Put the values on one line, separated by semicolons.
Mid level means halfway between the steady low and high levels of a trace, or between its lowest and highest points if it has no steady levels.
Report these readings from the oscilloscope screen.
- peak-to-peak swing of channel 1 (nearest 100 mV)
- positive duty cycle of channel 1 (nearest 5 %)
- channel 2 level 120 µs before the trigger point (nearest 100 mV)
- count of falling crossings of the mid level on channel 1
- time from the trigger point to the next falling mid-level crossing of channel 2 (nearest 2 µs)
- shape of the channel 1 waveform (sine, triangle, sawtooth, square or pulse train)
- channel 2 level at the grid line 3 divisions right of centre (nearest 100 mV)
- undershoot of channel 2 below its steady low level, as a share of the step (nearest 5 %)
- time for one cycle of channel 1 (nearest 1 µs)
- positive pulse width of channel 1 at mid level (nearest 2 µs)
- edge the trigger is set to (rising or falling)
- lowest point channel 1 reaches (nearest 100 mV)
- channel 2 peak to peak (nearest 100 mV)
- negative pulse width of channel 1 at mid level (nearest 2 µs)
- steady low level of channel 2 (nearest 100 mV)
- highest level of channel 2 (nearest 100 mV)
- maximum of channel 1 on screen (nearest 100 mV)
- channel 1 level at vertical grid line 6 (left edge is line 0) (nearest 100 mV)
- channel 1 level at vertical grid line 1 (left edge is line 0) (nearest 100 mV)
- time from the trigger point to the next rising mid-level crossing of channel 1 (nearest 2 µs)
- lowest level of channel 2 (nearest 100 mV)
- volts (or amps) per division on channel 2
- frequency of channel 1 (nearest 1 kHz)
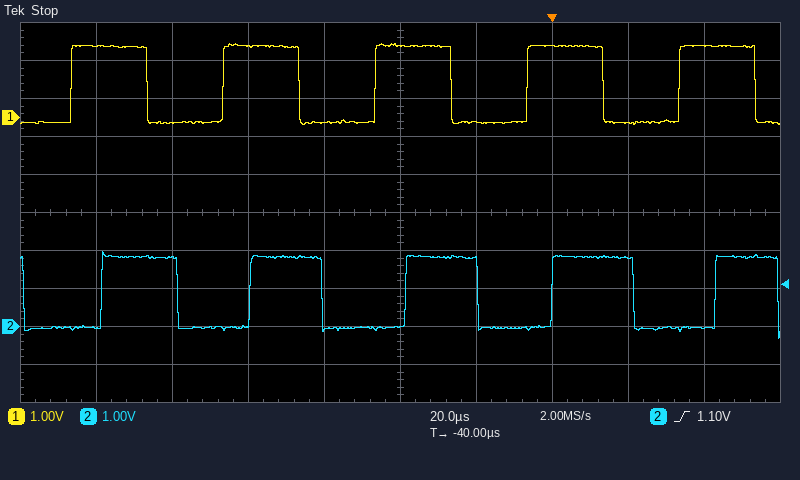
2.1 V; 50 %; 0.0 V; 5; 22 µs; square; 1.8 V; 15 %; 40 µs; 20 µs; rising; -200 mV; 2.3 V; 20 µs; 0.0 V; 2.0 V; 1.9 V; -100 mV; 1.9 V; 34 µs; -300 mV; 1 V; 25 kHz
